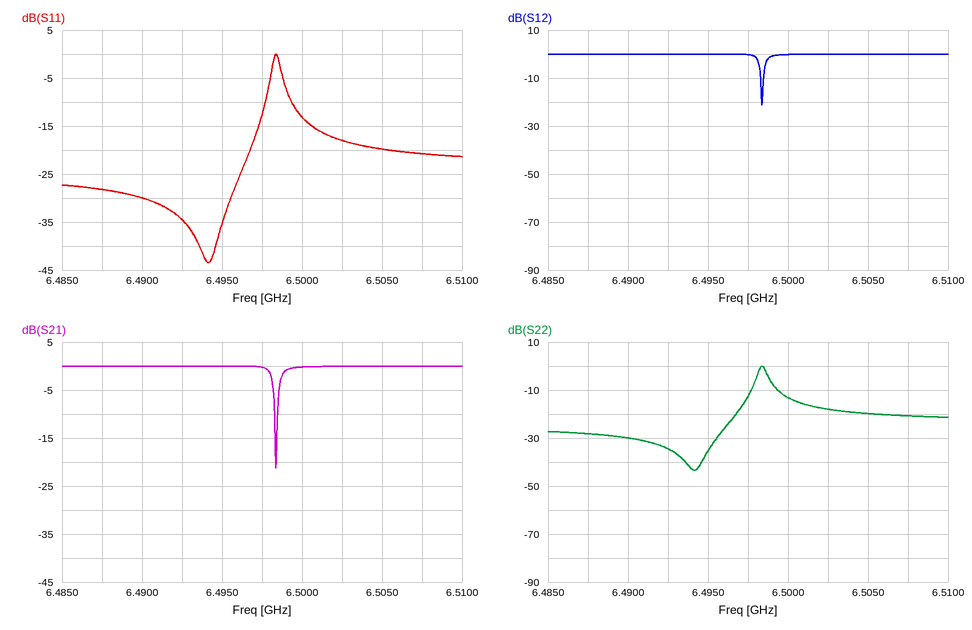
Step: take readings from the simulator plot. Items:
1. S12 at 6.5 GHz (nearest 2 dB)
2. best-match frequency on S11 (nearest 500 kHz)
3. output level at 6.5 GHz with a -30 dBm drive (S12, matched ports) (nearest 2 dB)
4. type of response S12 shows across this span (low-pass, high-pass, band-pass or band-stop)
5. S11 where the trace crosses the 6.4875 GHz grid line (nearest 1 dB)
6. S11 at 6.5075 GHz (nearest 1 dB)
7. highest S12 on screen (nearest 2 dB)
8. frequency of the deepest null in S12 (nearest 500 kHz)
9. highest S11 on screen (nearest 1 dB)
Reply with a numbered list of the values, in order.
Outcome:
1. 0 dB
2. 6.4940 GHz
3. -30 dBm
4. band-stop
5. -28 dB
6. -21 dB
7. 0 dB
8. 6.4985 GHz
9. 0 dB
